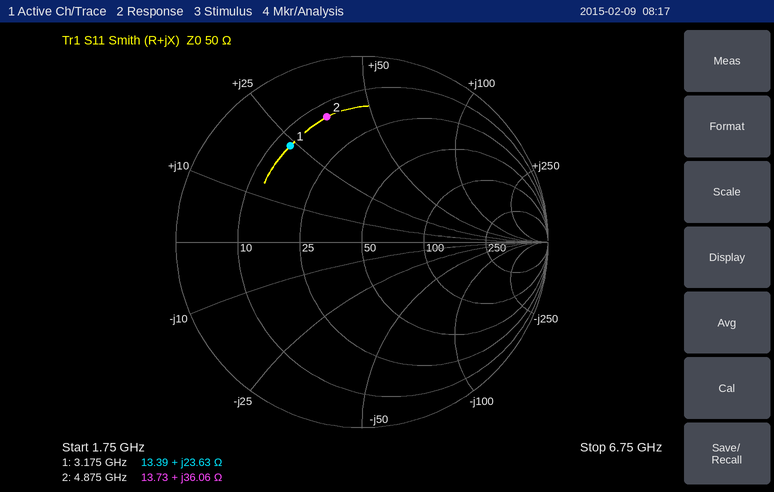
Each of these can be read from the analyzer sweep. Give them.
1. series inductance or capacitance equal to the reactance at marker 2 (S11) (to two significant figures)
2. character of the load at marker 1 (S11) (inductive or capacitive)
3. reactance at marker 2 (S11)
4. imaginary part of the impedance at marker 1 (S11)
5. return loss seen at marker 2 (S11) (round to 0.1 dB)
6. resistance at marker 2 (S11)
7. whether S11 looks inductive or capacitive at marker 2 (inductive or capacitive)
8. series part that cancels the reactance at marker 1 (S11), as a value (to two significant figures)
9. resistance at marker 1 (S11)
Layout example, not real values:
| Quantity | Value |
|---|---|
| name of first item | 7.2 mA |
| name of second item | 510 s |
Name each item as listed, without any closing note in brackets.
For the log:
| Quantity | Value |
|---|---|
| series inductance or capacitance equal to the reactance at marker 2 (S11) | 1.2 nH |
| character of the load at marker 1 (S11) | inductive |
| reactance at marker 2 | +36.06 Ω |
| imaginary part of the impedance at marker 1 | +23.63 Ω |
| return loss seen at marker 2 (S11) | 3.1 dB |
| resistance at marker 2 | 13.73 Ω |
| whether S11 looks inductive or capacitive at marker 2 | inductive |
| series part that cancels the reactance at marker 1 (S11), as a value | 2.1 pF |
| resistance at marker 1 | 13.39 Ω |
